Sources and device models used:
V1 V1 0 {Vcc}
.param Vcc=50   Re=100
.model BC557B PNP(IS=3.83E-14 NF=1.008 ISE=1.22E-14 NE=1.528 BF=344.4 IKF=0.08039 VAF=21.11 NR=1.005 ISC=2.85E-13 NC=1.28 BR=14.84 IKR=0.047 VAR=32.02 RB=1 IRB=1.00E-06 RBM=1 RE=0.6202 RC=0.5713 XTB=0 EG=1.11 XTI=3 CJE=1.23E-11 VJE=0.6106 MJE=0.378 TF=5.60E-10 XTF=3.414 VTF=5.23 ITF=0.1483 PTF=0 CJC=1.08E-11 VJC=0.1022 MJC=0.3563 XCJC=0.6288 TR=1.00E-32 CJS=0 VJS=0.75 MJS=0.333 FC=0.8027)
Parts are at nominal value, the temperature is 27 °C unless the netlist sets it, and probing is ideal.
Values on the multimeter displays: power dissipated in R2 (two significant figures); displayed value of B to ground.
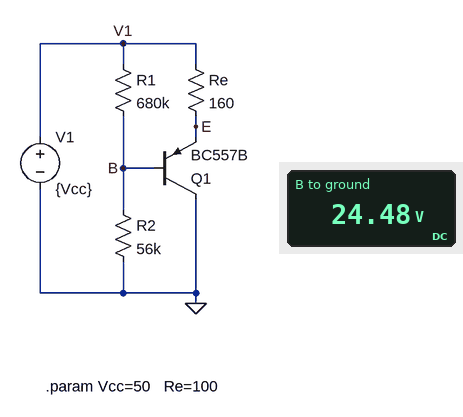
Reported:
11 mW
24.48 V
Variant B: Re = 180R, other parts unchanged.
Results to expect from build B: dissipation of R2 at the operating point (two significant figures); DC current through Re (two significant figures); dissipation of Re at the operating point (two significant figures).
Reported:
9.7 mW
140 mA
3.7 W
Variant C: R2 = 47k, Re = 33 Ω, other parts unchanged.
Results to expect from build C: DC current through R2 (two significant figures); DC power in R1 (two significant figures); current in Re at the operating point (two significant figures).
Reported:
820 µA
190 µW
320 mA
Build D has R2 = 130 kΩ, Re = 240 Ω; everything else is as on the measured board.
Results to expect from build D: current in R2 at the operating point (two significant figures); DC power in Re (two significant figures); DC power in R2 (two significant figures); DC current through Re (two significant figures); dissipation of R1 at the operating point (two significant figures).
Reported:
210 µA
2.0 W
5.7 mW
91 mA
760 µW
